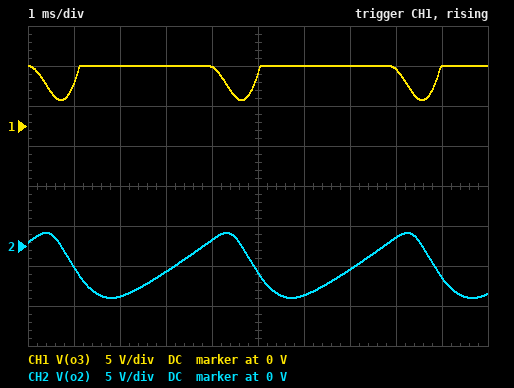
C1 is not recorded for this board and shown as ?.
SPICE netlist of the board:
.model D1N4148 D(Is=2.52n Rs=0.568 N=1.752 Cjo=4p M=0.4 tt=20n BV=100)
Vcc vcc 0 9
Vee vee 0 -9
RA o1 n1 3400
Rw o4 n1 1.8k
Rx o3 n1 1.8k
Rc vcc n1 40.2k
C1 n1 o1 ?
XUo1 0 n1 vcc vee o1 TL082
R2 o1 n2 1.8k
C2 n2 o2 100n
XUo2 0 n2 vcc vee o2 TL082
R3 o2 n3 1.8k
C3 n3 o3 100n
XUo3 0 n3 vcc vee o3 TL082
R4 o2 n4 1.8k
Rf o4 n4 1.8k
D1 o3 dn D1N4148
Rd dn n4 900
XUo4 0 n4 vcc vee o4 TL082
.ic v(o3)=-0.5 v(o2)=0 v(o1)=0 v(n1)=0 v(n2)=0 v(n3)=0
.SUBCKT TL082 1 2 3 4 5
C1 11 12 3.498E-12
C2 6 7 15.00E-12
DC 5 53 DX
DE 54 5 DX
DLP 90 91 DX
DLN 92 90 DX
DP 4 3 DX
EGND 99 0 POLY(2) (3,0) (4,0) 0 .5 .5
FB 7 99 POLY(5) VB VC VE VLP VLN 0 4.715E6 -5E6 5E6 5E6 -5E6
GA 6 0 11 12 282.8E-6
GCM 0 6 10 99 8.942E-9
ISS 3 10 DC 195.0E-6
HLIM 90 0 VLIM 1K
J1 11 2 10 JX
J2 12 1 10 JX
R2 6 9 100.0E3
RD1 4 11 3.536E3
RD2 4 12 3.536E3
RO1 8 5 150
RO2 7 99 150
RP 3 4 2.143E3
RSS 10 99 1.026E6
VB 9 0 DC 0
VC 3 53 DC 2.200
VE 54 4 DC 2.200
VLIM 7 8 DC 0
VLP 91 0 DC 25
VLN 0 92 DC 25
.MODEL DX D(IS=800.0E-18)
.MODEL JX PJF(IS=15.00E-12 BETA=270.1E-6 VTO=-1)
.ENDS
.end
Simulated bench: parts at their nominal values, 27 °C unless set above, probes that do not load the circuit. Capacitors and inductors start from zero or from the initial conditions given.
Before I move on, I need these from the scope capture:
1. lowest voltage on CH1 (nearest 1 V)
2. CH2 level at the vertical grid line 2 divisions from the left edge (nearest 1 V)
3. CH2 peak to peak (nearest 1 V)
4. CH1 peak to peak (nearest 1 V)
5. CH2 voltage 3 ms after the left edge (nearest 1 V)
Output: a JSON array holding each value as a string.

["3 V", "-6 V", "8 V", "4 V", "-3 V"]
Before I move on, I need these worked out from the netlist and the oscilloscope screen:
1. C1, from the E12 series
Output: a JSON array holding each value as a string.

["220 nF"]
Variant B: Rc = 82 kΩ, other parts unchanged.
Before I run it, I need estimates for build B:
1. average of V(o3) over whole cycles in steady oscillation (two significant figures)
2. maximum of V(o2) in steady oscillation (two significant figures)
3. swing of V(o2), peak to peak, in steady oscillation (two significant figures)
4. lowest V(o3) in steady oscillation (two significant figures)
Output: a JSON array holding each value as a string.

["7.3 V", "790 mV", "6.4 V", "5.4 V"]
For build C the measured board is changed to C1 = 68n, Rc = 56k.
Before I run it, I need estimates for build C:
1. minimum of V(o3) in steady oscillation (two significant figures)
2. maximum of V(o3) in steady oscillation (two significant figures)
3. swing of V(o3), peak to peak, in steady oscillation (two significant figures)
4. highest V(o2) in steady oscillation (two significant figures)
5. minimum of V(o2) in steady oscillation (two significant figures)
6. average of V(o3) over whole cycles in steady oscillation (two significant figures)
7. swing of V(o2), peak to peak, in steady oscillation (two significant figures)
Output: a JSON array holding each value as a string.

["-1.2 V", "870 mV", "2.1 V", "1.2 V", "-1.3 V", "-160 mV", "2.5 V"]
